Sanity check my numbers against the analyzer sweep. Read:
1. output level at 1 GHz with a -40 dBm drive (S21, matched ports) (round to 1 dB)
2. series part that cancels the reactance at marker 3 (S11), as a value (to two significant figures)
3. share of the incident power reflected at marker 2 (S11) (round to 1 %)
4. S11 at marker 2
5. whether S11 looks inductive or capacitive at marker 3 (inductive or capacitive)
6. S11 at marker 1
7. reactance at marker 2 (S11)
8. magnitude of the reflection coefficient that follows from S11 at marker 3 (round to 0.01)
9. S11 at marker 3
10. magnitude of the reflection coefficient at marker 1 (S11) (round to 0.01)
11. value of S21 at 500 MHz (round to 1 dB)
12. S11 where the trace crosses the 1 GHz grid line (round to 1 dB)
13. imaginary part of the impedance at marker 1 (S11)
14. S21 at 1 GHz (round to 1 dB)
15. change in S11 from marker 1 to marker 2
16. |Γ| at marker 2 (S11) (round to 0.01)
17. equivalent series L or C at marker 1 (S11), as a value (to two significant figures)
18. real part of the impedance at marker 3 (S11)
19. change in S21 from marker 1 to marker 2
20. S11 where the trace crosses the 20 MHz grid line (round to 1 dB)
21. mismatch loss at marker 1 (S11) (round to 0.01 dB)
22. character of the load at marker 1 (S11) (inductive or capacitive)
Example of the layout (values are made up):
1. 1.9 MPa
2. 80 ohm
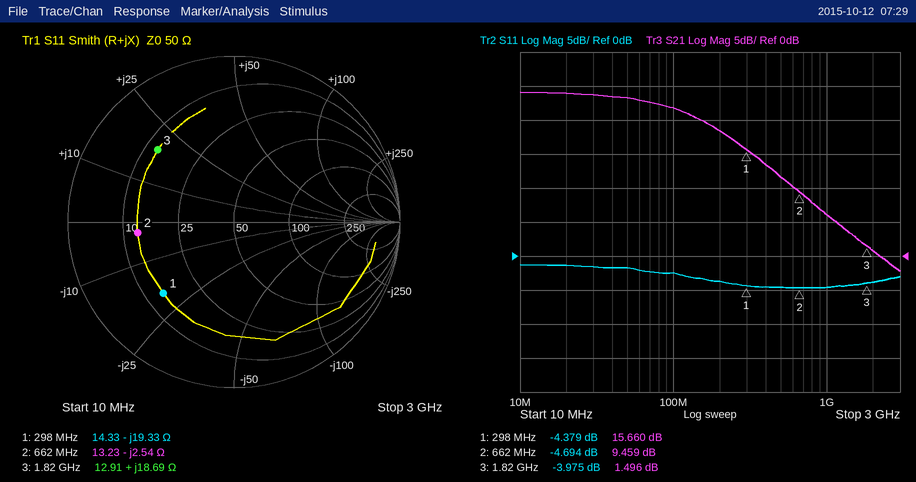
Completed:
1. -34 dBm
2. 4.7 pF
3. 34 %
4. -4.694 dB
5. inductive
6. -4.379 dB
7. -2.54 Ω
8. 0.63
9. -3.975 dB
10. 0.60
11. 12 dB
12. -5 dB
13. -19.33 Ω
14. 6 dB
15. -0.315 dB
16. 0.58
17. 28 pF
18. 12.91 Ω
19. -6.201 dB
20. -1 dB
21. 1.97 dB
22. capacitive
